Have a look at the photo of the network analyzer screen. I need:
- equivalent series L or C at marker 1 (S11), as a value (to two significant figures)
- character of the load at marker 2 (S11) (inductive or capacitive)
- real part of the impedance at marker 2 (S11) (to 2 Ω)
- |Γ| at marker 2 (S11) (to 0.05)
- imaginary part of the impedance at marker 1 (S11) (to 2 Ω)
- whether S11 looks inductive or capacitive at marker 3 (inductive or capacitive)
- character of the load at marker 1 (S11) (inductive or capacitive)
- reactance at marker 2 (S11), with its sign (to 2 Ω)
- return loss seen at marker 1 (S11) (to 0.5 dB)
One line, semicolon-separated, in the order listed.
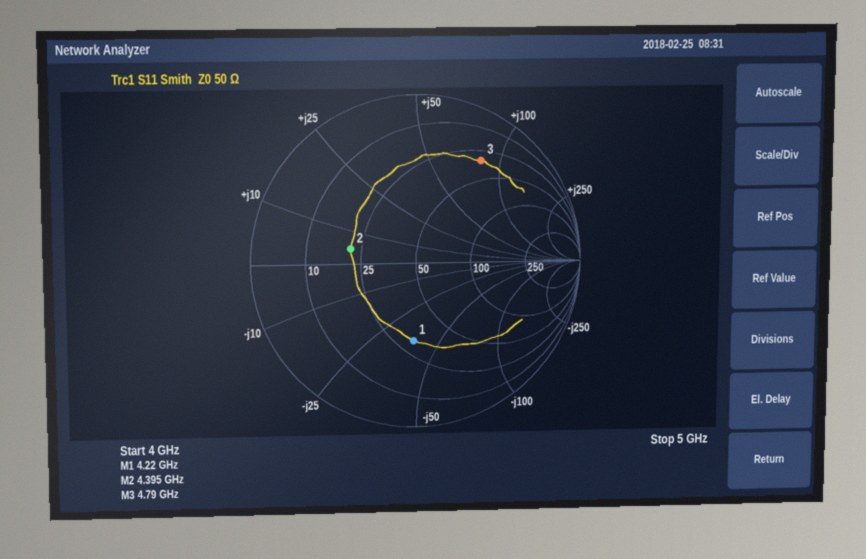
1.0 pF; inductive; 22 Ω; 0.40; -38 Ω; inductive; capacitive; +4 Ω; 6.5 dB
